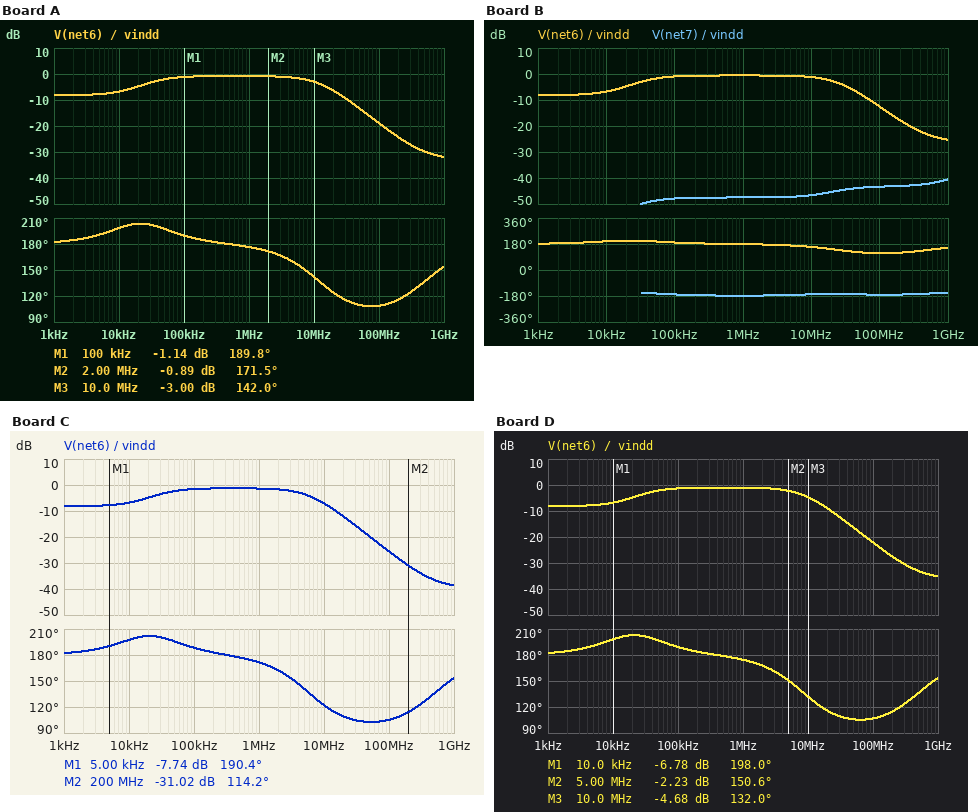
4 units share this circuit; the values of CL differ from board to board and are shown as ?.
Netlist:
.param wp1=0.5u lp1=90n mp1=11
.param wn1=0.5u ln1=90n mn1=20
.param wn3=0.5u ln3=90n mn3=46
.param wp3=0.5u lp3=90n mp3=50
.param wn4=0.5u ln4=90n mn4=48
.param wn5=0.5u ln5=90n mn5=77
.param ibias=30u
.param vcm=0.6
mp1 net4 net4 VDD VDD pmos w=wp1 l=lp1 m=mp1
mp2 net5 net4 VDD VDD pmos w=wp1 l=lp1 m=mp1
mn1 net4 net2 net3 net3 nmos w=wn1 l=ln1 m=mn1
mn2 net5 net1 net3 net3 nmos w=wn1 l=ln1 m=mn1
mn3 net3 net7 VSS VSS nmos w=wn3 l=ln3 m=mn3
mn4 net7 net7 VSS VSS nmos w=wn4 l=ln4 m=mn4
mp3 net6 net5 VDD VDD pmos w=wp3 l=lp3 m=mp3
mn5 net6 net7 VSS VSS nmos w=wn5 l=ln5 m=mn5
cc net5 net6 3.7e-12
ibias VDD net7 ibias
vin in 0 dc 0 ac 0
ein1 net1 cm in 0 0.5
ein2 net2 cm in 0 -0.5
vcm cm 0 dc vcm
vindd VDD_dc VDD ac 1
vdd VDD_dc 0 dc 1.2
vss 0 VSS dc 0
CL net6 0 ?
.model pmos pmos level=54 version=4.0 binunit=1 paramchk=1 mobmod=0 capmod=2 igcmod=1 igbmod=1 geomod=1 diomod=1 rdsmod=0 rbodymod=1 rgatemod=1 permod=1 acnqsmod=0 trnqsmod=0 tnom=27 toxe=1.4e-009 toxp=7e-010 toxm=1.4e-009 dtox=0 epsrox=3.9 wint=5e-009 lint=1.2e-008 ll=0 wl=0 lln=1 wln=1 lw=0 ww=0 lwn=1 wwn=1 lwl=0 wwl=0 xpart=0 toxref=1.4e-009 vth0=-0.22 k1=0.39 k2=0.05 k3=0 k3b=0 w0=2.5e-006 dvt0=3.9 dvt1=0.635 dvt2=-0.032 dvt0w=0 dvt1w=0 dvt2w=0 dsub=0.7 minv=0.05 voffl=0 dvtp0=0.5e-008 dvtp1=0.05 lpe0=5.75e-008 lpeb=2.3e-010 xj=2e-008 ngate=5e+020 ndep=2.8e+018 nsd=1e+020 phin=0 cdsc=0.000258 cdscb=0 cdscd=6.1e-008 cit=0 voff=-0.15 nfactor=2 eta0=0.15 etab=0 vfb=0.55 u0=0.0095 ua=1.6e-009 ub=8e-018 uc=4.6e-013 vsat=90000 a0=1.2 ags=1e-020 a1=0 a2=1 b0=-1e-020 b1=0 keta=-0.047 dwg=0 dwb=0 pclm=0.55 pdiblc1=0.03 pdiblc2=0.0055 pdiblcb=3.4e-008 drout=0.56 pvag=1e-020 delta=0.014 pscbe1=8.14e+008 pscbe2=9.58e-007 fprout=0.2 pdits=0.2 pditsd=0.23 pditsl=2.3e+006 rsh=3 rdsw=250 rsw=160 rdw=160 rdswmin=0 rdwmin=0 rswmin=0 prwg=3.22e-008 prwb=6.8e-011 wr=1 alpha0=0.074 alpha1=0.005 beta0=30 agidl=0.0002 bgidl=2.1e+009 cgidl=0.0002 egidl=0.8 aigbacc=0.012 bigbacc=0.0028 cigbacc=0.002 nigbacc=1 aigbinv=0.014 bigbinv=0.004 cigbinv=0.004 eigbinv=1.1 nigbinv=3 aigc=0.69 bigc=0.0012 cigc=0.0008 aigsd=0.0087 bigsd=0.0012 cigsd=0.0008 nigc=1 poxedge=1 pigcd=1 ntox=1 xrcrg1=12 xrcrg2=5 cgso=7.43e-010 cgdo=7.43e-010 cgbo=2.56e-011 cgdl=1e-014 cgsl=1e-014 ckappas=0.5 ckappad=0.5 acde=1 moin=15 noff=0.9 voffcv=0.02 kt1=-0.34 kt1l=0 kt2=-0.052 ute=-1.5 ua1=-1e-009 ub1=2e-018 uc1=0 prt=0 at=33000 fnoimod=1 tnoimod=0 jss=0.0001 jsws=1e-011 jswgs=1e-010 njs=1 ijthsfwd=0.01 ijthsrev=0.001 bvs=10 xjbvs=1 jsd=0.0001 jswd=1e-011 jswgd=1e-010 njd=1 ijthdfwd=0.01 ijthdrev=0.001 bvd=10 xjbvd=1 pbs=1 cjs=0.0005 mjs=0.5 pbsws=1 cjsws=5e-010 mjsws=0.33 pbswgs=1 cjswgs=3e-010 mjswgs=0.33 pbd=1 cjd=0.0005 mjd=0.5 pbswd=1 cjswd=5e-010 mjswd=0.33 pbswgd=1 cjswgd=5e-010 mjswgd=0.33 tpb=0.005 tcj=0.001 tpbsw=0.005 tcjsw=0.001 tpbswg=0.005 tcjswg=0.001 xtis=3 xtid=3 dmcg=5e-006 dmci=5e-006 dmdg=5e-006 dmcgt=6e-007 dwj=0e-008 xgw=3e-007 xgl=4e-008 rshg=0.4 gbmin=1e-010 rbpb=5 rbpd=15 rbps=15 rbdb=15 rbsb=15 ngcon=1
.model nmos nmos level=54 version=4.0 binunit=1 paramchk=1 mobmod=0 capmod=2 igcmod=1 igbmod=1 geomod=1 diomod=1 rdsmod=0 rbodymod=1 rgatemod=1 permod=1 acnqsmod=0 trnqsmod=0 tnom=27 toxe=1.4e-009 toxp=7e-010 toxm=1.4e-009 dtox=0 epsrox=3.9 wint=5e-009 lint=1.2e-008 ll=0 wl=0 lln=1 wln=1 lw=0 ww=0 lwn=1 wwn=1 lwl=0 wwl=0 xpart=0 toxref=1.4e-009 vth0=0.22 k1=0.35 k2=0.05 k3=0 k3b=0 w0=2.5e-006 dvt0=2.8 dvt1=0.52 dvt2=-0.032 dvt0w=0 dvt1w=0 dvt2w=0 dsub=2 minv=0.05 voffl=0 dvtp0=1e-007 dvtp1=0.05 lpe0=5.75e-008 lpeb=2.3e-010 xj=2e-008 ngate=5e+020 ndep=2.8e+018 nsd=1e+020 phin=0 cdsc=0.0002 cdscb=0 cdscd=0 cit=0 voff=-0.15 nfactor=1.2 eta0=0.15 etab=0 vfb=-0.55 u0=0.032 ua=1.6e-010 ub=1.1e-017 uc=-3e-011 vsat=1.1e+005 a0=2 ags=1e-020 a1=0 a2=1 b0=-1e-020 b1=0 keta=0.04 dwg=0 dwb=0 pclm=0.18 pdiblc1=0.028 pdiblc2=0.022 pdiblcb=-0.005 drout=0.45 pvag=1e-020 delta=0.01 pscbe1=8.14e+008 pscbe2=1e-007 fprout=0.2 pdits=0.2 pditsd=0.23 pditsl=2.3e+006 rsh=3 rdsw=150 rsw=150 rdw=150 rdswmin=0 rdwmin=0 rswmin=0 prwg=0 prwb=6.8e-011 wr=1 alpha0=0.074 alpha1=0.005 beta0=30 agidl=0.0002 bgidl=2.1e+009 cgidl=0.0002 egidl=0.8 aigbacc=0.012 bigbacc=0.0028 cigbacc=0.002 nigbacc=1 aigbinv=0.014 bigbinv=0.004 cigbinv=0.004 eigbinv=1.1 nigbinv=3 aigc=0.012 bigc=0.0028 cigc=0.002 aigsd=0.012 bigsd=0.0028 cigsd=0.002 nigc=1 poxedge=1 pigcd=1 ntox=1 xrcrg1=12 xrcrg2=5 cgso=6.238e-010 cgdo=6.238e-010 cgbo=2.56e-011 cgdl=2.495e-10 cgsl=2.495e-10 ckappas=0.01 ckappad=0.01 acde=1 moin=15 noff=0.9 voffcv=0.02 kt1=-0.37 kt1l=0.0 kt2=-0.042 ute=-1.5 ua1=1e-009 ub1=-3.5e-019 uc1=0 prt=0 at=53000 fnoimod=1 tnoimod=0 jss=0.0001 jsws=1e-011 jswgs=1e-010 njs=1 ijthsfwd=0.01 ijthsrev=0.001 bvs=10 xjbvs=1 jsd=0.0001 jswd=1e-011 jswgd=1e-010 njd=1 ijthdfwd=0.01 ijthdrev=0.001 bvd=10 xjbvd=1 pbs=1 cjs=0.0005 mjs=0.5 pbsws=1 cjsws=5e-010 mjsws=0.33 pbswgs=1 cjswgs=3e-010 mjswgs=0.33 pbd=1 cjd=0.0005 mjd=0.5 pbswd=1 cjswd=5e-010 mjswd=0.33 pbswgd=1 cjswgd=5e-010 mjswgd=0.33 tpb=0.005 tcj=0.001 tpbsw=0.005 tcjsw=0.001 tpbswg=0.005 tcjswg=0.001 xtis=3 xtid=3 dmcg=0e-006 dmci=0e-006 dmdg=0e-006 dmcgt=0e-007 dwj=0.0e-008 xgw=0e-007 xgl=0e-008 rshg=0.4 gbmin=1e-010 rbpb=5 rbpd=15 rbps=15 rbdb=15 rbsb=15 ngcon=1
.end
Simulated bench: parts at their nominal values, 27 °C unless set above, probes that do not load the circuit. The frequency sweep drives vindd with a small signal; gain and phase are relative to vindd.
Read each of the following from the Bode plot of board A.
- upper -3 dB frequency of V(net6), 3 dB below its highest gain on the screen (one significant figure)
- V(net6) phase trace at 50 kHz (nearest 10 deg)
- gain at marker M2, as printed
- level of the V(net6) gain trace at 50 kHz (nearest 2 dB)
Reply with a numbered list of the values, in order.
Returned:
1. 10 MHz
2. 200 deg
3. -0.89 dB
4. -2 dB
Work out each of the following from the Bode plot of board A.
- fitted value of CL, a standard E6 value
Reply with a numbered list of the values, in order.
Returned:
1. 15 pF
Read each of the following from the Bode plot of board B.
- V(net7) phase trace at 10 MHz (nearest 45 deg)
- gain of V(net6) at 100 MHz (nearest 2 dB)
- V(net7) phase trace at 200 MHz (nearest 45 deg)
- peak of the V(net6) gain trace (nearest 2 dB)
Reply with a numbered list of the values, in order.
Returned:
1. -180 deg
2. -12 dB
3. -180 deg
4. 0 dB
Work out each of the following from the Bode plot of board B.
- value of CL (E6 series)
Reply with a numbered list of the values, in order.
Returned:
1. 6.8 pF
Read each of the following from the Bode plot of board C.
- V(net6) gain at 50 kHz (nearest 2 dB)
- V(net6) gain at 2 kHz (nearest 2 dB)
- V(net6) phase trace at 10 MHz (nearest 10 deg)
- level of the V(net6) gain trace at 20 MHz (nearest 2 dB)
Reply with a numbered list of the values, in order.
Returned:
1. -2 dB
2. -8 dB
3. 120 deg
4. -12 dB
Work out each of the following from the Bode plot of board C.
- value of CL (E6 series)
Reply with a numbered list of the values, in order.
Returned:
1. 33 pF
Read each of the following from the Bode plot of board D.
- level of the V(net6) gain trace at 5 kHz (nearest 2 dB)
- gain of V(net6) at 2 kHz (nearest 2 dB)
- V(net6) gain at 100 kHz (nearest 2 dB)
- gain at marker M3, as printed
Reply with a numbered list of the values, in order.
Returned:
1. -8 dB
2. -8 dB
3. -2 dB
4. -4.68 dB
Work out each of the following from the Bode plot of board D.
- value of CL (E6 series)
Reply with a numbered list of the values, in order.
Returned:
1. 22 pF
